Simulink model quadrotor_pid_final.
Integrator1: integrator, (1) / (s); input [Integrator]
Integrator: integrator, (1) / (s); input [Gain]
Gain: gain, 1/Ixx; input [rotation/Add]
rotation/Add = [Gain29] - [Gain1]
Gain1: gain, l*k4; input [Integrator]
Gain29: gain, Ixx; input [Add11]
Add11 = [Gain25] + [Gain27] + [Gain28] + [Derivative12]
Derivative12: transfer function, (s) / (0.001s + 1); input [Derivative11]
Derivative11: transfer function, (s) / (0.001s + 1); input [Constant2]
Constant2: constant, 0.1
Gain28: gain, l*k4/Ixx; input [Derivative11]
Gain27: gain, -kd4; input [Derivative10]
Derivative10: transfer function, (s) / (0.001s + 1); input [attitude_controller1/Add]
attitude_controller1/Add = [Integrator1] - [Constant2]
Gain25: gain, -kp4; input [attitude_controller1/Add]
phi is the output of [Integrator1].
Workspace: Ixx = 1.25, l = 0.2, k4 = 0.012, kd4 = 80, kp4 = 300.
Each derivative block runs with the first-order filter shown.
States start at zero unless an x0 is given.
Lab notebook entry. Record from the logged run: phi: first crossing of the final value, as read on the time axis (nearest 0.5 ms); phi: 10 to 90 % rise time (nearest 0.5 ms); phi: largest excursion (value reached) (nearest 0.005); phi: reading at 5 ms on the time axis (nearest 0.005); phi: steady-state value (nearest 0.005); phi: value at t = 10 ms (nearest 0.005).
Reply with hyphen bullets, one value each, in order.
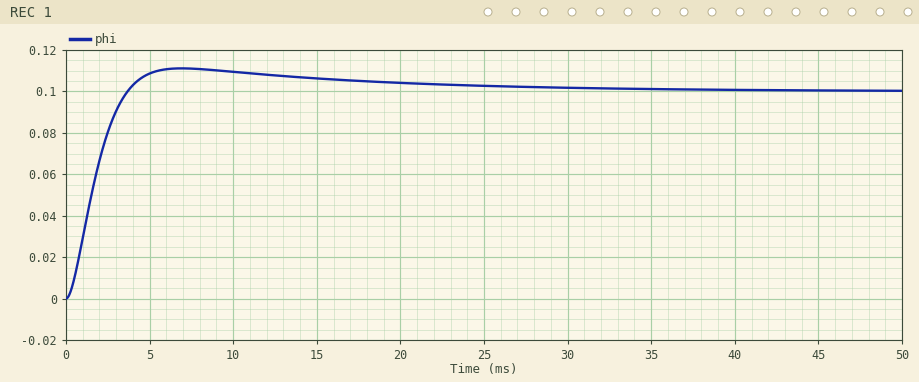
- 3.5 ms
- 2.5 ms
- 0.110
- 0.110
- 0.100
- 0.110
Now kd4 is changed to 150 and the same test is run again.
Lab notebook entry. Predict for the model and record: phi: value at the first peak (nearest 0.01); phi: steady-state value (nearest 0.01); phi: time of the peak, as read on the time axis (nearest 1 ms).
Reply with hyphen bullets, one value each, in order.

- 0.12
- 0.10
- 6 ms
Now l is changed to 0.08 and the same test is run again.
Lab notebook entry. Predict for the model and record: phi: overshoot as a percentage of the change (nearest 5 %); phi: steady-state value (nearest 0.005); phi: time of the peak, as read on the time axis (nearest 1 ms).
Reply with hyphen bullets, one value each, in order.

- 10 %
- 0.100
- 7 ms
